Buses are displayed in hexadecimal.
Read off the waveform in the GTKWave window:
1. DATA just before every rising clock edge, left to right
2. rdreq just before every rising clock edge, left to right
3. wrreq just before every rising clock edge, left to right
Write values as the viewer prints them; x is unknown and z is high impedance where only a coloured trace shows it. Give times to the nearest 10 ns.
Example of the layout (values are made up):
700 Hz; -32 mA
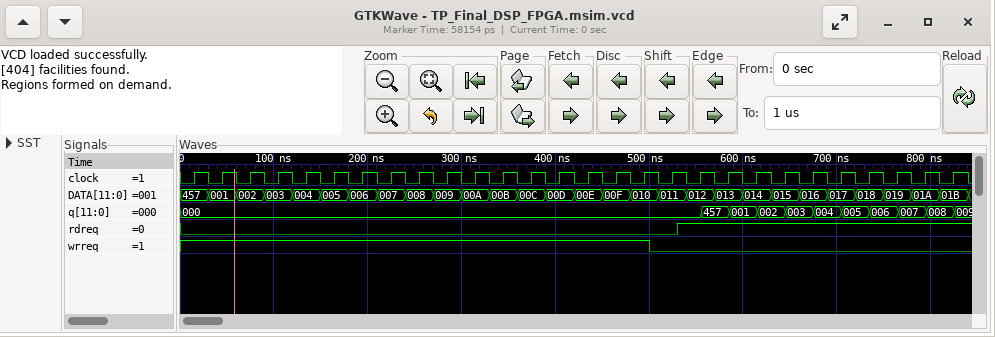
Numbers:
457, 001, 002, 003, 004, 005, 006, 007, 008, 009, 00A, 00B, 00C, 00D, 00E, 00F, 010, 011, 012, 013, 014, 015, 016, 017, 018, 019, 01A, 01B; 0 0 0 0 0 0 0 0 0 0 0 0 0 0 0 0 0 0 1 1 1 1 1 1 1 1 1 1; 1 1 1 1 1 1 1 1 1 1 1 1 1 1 1 1 1 0 0 0 0 0 0 0 0 0 0 0
